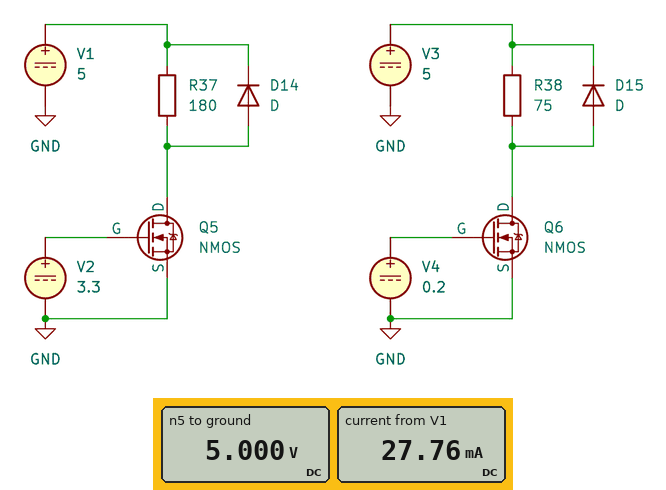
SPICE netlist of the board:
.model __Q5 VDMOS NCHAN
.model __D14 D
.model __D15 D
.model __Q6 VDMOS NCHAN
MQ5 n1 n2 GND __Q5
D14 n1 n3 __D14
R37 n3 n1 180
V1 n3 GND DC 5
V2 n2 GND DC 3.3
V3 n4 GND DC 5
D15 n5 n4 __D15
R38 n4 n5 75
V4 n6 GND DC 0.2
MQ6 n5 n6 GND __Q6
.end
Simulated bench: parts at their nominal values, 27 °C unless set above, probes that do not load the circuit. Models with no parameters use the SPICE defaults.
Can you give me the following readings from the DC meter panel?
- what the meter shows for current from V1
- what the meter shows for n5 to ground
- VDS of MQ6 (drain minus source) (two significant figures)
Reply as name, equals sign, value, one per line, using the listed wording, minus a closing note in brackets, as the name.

what the meter shows for current from V1 = 27.76 mA
what the meter shows for n5 to ground = 5.000 V
VDS of MQ6 (drain minus source) = 5.0 V
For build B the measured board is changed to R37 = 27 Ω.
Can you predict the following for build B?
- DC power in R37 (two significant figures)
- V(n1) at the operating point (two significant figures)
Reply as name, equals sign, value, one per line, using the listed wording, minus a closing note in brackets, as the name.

DC power in R37 = 920 mW
V(n1) at the operating point = 18 mV
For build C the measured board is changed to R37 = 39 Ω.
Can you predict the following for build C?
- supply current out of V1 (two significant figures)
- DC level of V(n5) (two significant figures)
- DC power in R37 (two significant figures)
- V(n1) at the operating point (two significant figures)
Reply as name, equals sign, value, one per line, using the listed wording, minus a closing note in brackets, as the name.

supply current out of V1 = 130 mA
DC level of V(n5) = 5.0 V
DC power in R37 = 640 mW
V(n1) at the operating point = 12 mV
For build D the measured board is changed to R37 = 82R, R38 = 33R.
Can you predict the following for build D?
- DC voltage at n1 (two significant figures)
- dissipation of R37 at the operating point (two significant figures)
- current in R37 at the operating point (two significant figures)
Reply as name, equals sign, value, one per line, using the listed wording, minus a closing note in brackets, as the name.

DC voltage at n1 = 5.8 mV
dissipation of R37 at the operating point = 300 mW
current in R37 at the operating point = 61 mA
